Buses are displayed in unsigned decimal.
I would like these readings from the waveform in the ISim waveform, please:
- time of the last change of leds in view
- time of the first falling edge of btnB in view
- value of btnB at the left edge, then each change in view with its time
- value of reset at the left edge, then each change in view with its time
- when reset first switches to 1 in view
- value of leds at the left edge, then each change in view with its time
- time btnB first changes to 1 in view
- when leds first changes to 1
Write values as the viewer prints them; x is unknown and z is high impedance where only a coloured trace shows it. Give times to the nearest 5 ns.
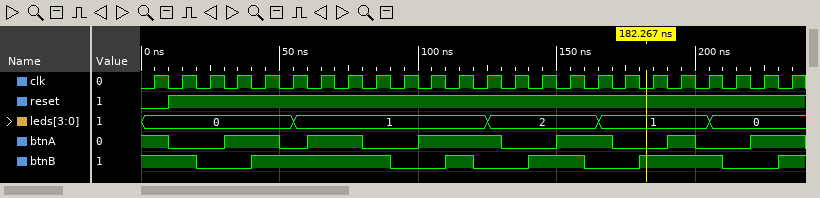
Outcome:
205 ns
20 ns
1, 0 at 20 ns, 1 at 40 ns, 0 at 90 ns, 1 at 110 ns, 0 at 120 ns, 1 at 140 ns, 0 at 160 ns, 1 at 180 ns, 0 at 210 ns, 1 at 230 ns
0, 1 at 10 ns
10 ns
0, 1 at 55 ns, 2 at 125 ns, 1 at 165 ns, 0 at 205 ns
40 ns
55 ns
